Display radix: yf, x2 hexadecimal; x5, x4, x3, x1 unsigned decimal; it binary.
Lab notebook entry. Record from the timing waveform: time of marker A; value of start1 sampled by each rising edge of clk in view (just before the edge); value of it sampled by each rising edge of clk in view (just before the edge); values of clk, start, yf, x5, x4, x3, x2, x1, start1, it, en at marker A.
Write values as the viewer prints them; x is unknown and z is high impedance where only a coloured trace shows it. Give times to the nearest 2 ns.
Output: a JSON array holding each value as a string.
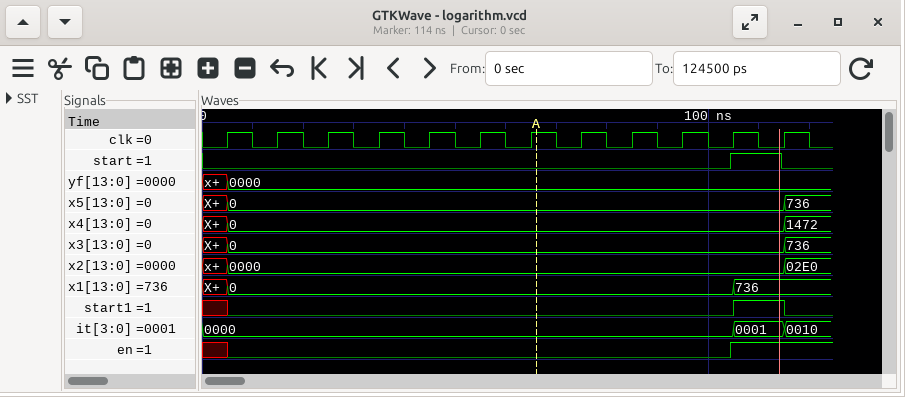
["66 ns", "x 0 0 0 0 0 0 0 0 0 0 1", "0000, 0000, 0000, 0000, 0000, 0000, 0000, 0000, 0000, 0000, 0000, 0001", "clk=1, start=0, yf=0000, x5=0, x4=0, x3=0, x2=0000, x1=0, start1=0, it=0000, en=0"]
